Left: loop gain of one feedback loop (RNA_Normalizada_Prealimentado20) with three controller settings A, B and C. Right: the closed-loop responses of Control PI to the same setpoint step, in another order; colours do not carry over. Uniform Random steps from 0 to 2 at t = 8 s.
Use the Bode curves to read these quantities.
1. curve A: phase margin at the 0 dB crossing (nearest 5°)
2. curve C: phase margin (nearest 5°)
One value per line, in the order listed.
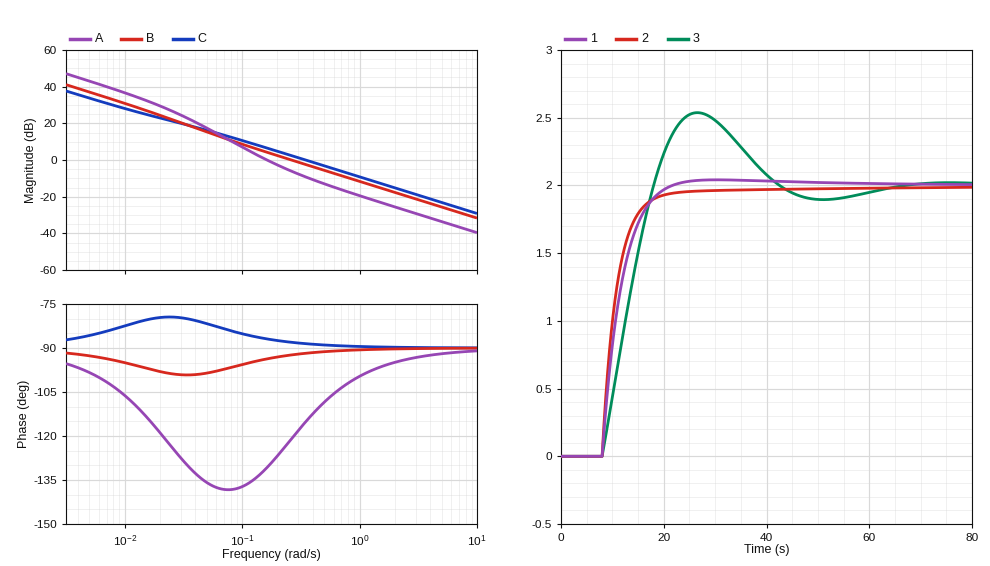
50°
90°
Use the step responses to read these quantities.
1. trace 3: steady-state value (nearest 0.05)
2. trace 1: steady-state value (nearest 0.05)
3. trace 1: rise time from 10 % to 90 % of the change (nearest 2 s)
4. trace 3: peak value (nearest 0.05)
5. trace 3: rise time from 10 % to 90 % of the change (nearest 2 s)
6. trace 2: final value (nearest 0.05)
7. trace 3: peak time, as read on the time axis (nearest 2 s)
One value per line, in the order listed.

2.00
2.00
8 s
2.55
8 s
2.00
26 s
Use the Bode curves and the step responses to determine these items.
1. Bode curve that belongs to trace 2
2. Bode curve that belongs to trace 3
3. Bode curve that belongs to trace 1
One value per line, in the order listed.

C
A
B
